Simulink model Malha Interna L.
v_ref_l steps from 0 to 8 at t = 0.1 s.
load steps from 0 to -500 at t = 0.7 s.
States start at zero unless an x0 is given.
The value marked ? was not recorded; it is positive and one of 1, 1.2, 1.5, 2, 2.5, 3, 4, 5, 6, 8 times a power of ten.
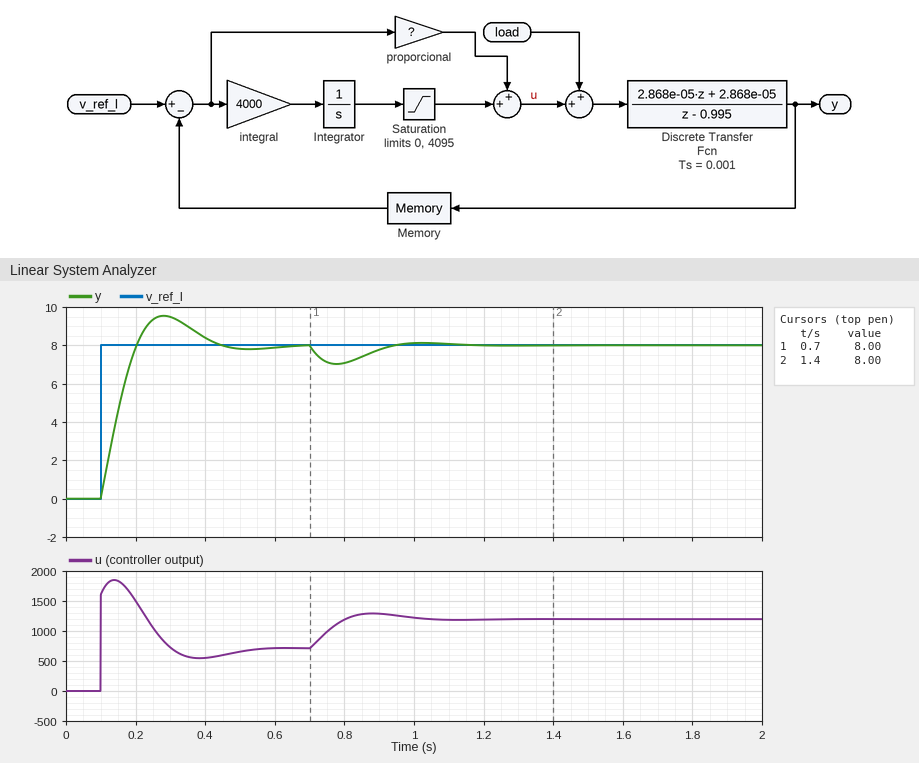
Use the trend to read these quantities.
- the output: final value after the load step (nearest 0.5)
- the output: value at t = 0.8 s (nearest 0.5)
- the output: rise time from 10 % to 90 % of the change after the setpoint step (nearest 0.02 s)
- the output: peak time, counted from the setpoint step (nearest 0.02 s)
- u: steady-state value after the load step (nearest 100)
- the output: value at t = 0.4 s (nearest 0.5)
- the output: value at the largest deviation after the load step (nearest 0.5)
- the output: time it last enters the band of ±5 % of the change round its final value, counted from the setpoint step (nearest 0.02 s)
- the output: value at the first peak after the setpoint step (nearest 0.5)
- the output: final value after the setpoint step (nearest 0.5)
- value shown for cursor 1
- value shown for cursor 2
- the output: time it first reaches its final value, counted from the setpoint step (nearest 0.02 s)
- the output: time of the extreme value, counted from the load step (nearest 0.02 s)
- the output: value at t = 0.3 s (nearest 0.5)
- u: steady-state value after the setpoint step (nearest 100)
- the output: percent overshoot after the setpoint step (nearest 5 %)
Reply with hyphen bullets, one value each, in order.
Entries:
- 8.0
- 7.0
- 0.08 s
- 0.18 s
- 1200
- 8.5
- 7.0
- 0.30 s
- 9.5
- 8.0
- 8.00
- 8.00
- 0.10 s
- 0.08 s
- 9.5
- 700
- 20 %
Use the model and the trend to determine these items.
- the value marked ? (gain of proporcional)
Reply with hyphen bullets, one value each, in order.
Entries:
- 200
